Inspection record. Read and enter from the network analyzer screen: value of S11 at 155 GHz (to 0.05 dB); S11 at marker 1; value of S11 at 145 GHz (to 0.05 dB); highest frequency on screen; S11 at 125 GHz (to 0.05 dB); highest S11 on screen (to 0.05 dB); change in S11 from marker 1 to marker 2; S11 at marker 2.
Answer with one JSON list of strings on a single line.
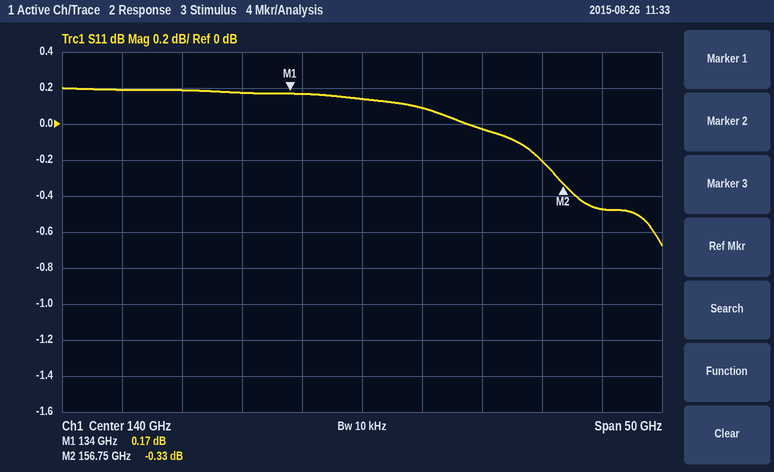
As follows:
["-0.20 dB", "0.17 dB", "0.10 dB", "165 GHz", "0.20 dB", "0.20 dB", "-0.50 dB", "-0.33 dB"]
